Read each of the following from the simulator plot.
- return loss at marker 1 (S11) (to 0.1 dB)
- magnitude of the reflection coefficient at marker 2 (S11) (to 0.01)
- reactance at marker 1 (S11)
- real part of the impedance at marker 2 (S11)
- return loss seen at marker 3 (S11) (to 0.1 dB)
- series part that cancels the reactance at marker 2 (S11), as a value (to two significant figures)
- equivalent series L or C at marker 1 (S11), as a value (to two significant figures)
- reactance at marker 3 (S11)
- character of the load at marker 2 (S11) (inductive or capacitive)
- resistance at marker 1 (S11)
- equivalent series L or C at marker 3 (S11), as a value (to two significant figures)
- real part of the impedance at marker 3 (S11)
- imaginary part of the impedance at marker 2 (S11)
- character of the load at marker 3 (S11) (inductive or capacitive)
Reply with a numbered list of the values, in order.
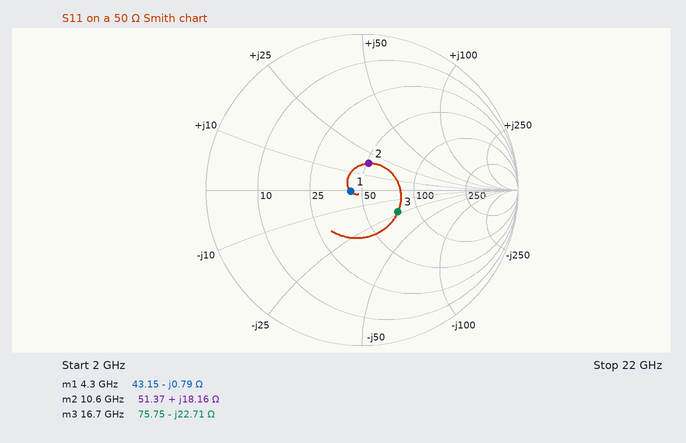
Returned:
1. 22.6 dB
2. 0.18
3. -0.79 Ω
4. 51.37 Ω
5. 11.4 dB
6. 830 fF
7. 47 pF
8. -22.71 Ω
9. inductive
10. 43.15 Ω
11. 420 fF
12. 75.75 Ω
13. +18.16 Ω
14. capacitive
